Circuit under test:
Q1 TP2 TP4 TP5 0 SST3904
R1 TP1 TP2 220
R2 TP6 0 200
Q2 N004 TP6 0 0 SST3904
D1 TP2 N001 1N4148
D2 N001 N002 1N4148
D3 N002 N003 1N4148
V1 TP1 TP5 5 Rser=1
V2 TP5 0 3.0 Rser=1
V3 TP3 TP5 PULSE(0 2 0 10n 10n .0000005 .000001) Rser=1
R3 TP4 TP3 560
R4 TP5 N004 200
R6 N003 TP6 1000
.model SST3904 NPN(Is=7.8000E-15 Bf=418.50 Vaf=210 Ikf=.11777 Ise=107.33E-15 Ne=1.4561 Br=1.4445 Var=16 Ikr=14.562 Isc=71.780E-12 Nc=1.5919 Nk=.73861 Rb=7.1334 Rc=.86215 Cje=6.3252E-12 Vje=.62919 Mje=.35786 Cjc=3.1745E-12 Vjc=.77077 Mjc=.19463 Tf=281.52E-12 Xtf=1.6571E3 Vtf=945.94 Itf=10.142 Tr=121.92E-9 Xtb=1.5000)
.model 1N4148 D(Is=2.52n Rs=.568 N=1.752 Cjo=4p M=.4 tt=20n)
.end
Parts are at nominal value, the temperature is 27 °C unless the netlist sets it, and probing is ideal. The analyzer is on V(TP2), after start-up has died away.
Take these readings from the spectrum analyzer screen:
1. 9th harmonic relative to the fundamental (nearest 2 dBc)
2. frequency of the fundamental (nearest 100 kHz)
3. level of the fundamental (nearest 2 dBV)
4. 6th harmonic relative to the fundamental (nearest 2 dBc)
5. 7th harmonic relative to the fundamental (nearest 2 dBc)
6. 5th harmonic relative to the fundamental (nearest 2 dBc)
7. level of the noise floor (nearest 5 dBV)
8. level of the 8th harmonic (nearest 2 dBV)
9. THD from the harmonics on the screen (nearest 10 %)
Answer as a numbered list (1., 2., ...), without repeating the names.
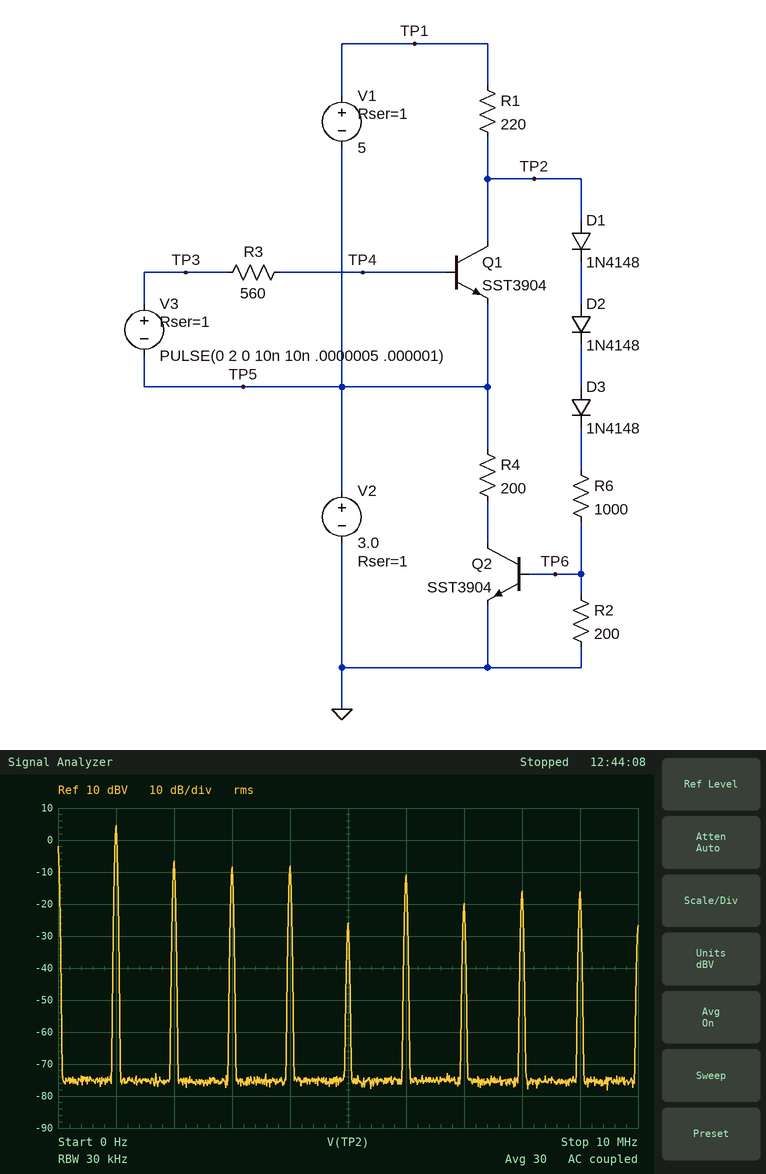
1. -20 dBc
2. 1.0 MHz
3. 4 dBV
4. -16 dBc
5. -24 dBc
6. -30 dBc
7. -75 dBV
8. -16 dBV
9. 50 %
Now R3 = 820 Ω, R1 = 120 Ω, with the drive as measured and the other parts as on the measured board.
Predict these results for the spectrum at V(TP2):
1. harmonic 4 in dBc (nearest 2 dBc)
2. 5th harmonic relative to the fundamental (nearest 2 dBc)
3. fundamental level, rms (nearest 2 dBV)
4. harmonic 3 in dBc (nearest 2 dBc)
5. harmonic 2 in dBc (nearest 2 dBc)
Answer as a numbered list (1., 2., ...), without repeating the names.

1. -14 dBc
2. -20 dBc
3. 6 dBV
4. -12 dBc
5. -14 dBc
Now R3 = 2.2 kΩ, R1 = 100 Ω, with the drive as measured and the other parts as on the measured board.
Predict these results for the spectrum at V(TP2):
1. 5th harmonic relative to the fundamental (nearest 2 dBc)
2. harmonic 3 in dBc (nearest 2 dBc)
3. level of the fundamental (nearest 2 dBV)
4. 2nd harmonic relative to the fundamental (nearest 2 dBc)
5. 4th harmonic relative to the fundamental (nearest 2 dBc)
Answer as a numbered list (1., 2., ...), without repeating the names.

1. -16 dBc
2. -10 dBc
3. 6 dBV
4. -28 dBc
5. -28 dBc
